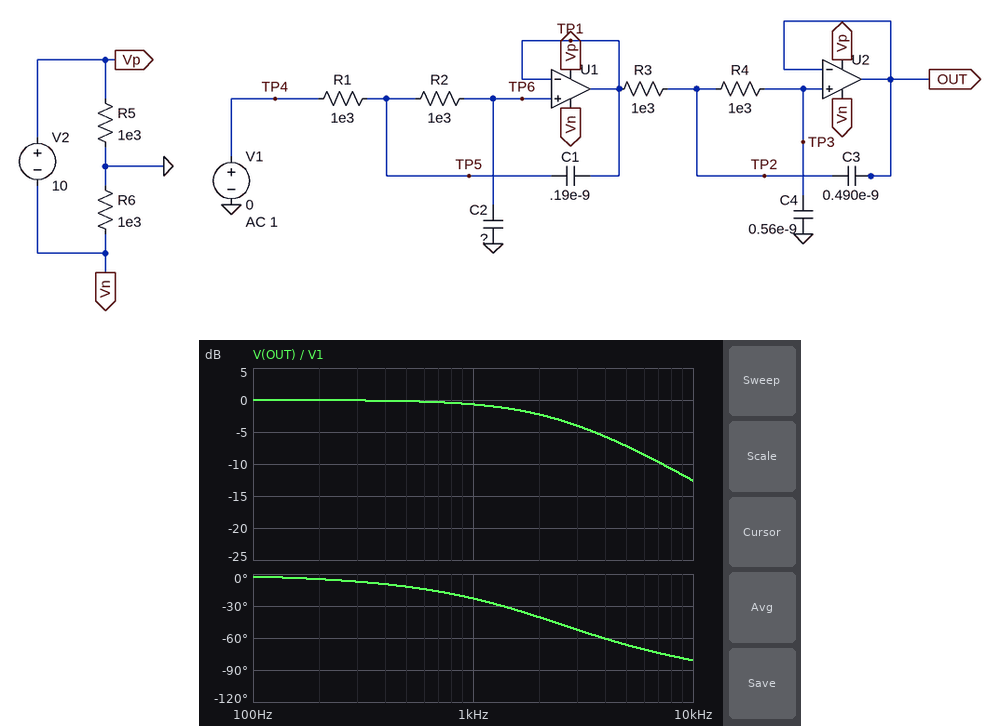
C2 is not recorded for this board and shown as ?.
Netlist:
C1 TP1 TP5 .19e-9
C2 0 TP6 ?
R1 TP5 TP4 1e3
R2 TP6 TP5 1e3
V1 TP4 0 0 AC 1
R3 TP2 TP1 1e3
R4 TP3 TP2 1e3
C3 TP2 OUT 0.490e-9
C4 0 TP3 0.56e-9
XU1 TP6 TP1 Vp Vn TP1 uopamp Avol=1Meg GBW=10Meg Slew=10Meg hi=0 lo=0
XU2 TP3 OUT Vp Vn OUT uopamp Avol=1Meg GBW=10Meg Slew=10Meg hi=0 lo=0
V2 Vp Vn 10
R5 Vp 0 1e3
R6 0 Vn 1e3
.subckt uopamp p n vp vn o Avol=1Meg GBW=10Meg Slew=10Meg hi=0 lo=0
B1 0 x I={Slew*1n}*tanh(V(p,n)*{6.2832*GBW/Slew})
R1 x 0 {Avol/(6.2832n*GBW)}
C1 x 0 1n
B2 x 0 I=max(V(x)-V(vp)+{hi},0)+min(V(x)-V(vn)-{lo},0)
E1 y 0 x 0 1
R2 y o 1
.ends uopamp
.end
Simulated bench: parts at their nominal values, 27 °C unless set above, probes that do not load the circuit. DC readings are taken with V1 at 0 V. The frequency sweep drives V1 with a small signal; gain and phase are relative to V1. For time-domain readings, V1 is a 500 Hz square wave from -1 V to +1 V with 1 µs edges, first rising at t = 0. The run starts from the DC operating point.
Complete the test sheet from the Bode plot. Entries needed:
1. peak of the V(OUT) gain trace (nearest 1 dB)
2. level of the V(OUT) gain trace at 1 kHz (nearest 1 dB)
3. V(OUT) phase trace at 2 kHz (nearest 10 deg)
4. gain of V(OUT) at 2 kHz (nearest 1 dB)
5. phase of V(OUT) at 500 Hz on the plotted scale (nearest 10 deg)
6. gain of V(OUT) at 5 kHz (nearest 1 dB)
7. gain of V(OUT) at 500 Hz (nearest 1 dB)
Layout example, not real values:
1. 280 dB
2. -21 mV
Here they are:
1. 0 dB
2. -1 dB
3. -40 deg
4. -2 dB
5. -10 deg
6. -7 dB
7. 0 dB
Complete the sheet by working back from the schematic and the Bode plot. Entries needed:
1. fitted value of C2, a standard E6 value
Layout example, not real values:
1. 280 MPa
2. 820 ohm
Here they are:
1. 33 nF
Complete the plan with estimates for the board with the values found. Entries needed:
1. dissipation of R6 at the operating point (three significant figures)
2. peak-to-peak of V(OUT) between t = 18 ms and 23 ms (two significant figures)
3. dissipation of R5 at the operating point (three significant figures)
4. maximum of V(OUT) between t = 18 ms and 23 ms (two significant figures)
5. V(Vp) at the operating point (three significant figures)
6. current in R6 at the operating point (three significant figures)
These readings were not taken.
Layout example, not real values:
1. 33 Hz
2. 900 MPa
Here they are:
1. 25.0 mW
2. 2.0 V
3. 25.0 mW
4. 1.0 V
5. 5.00 V
6. 5.00 mA
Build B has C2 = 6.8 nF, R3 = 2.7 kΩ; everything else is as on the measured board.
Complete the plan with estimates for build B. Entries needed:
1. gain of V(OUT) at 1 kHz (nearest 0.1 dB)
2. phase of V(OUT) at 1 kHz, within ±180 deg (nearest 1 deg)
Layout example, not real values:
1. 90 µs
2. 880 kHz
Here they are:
1. 0 dB
2. -6 deg
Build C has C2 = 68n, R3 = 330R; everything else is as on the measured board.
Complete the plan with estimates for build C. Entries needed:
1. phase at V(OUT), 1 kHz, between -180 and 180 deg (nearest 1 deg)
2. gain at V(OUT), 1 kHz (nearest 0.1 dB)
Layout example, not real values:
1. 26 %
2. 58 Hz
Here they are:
1. -41 deg
2. -2.4 dB
